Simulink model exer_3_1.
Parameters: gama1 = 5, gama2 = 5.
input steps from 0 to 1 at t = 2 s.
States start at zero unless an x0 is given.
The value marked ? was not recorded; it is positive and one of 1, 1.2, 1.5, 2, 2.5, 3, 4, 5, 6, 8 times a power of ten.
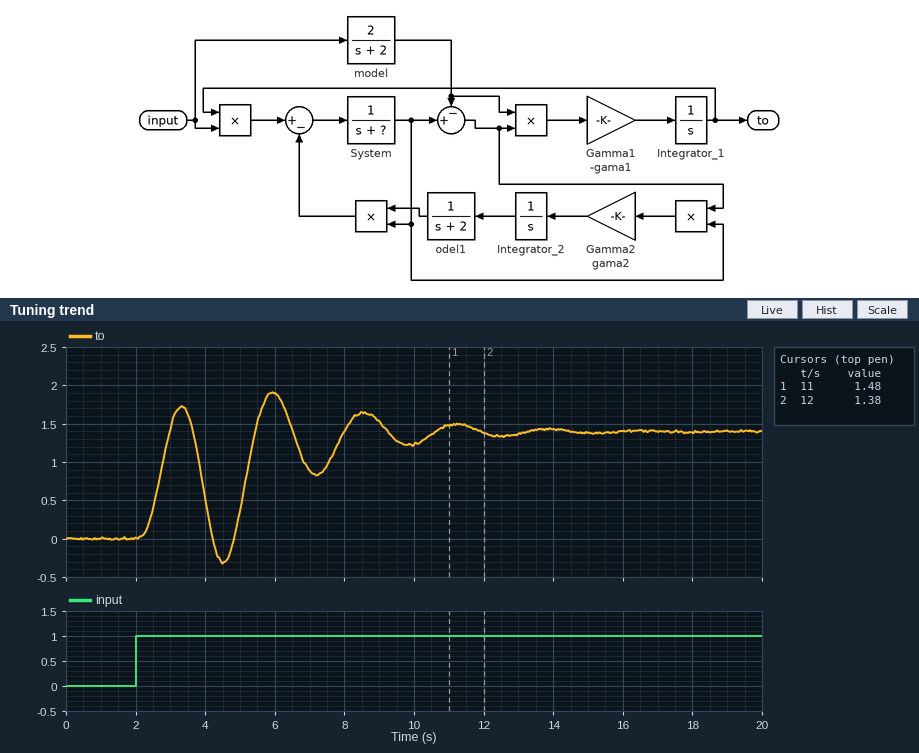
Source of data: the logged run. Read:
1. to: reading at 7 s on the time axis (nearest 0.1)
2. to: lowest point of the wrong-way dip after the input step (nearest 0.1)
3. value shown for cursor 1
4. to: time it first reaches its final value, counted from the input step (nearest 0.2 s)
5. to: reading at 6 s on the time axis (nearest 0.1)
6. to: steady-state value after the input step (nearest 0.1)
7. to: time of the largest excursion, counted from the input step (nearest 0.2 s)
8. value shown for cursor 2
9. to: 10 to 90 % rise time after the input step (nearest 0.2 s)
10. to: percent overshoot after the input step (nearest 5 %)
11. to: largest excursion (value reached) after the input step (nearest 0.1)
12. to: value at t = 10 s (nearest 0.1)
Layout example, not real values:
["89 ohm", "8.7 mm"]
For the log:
["0.9", "-0.3", "1.48", "1.0 s", "1.9", "1.4", "4.0 s", "1.38", "0.6 s", "35 %", "1.9", "1.2"]
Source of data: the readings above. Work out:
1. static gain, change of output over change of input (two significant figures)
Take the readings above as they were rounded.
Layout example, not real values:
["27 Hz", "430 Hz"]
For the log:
["1.4"]
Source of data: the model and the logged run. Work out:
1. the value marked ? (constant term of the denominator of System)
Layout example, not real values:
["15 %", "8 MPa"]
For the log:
["0.4"]
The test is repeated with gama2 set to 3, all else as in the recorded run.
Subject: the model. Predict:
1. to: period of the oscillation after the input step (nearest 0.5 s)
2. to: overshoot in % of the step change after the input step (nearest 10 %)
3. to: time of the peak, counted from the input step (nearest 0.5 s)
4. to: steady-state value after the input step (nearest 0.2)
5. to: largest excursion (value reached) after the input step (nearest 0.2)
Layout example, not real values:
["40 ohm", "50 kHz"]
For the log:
["2.5 s", "60 %", "1.5 s", "1.0", "1.8"]
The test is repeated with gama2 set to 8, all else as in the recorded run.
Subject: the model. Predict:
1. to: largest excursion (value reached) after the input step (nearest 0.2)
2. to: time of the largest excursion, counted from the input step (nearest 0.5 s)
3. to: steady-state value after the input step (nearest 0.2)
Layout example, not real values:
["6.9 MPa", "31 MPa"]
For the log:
["2.2", "4.0 s", "1.8"]
